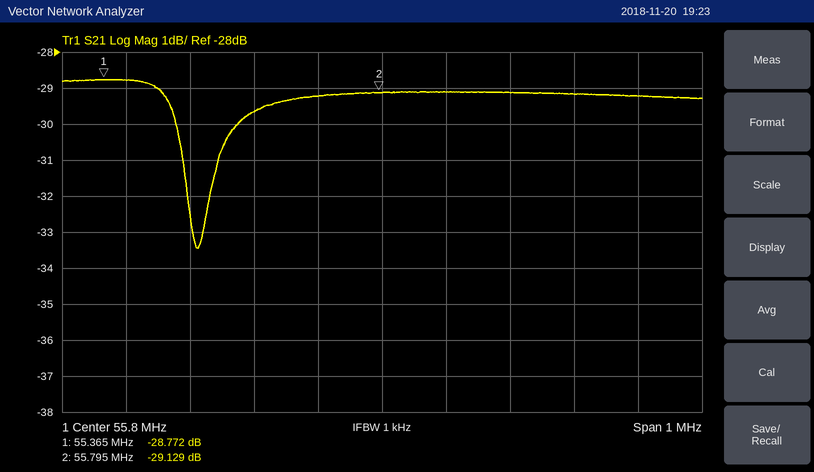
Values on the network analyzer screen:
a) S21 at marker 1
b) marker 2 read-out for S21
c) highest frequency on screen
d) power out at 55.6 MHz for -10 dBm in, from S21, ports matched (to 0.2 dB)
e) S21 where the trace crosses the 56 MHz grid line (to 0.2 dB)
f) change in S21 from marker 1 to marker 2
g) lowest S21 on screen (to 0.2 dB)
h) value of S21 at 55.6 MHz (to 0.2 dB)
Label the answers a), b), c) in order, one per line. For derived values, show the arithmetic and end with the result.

a) -28.772 dB
b) -29.129 dB
c) 56.3 MHz
d) -10 dBm + (-29.6 dB) = -39.6 dBm
e) -29.2 dB
f) -29.129 − (-28.772) = -0.357 dB
g) -33.4 dB
h) -29.6 dB
